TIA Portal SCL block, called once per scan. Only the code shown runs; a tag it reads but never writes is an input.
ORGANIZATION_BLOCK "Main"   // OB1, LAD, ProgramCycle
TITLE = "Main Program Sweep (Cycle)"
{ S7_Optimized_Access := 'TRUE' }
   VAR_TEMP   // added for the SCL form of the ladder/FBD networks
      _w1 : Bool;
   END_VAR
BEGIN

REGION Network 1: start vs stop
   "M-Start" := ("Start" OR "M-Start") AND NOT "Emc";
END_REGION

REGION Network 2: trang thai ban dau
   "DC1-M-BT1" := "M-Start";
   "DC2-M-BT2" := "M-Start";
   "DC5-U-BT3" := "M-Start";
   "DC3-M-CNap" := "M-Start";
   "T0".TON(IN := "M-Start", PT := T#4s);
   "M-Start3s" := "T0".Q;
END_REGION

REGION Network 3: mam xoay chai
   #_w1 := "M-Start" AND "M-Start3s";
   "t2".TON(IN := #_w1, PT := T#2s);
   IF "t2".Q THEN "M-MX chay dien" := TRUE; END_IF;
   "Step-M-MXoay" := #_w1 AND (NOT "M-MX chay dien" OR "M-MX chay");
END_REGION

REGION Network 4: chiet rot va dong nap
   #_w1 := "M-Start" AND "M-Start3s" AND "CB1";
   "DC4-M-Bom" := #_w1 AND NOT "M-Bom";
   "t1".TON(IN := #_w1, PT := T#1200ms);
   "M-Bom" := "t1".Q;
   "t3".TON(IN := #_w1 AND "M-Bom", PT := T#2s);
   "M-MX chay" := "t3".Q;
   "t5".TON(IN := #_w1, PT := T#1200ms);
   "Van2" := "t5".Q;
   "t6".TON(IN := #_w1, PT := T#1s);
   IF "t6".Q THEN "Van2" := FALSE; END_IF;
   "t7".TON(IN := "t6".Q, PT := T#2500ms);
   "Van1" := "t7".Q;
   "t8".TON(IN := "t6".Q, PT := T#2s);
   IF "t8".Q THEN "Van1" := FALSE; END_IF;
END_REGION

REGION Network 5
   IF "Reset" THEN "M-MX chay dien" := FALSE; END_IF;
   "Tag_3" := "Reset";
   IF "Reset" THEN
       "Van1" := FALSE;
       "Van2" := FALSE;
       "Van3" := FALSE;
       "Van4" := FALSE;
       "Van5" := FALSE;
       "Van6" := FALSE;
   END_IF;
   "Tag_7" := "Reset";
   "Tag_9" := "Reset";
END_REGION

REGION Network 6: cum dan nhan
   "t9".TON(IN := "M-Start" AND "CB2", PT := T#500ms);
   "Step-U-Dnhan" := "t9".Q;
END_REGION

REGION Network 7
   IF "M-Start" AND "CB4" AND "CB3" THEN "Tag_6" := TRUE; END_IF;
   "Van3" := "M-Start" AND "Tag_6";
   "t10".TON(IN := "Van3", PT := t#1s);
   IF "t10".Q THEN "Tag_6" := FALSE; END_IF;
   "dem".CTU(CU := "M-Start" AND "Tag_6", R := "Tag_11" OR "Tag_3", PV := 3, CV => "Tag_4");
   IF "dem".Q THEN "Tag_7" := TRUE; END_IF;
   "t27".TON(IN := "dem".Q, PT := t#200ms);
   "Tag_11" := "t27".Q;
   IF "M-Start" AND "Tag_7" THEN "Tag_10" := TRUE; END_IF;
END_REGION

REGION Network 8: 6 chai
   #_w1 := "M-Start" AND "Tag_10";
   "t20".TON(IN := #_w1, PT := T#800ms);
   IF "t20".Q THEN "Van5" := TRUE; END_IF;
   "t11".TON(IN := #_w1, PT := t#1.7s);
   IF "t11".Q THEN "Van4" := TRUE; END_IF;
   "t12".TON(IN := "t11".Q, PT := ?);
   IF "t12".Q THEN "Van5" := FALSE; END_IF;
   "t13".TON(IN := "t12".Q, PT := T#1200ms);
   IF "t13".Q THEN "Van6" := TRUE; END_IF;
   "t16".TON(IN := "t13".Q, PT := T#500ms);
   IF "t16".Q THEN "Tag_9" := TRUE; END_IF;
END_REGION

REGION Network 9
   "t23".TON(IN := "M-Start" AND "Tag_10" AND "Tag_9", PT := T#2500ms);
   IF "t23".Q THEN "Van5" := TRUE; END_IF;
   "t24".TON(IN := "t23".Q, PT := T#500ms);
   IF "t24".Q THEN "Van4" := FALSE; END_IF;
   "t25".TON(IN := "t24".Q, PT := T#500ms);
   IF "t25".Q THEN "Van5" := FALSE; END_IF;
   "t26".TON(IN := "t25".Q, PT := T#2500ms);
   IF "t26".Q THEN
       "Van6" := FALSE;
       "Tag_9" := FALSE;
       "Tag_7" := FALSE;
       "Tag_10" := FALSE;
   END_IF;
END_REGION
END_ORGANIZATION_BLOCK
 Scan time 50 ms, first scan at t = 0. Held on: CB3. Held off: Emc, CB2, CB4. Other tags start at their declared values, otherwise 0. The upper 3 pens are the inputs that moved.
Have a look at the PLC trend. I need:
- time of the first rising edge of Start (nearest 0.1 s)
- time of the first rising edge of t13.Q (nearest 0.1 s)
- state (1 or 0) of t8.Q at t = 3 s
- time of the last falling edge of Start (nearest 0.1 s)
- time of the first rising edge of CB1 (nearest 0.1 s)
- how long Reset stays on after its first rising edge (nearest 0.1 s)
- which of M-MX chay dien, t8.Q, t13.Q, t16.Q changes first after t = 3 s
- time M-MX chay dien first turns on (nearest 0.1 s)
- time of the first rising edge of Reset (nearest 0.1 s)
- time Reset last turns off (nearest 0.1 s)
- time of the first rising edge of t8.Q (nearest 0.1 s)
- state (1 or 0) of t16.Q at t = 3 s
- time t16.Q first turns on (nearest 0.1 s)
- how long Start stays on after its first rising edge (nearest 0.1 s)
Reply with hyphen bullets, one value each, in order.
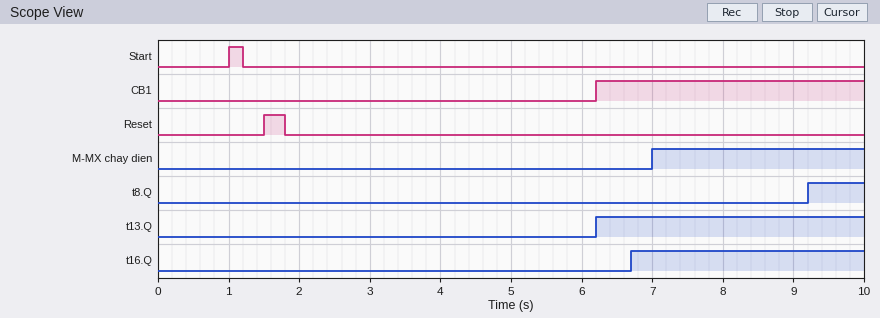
- 1.0 s
- 6.2 s
- 0
- 1.2 s
- 6.2 s
- 0.3 s
- t13.Q
- 7.0 s
- 1.5 s
- 1.8 s
- 9.2 s
- 0
- 6.7 s
- 0.2 s
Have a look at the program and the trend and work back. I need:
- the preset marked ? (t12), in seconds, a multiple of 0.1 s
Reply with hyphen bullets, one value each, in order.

- 1.8 s
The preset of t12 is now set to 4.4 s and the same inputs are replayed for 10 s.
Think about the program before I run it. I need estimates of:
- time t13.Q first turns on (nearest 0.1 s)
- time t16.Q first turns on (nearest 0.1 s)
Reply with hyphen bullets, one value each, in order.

- 8.8 s
- 9.3 s
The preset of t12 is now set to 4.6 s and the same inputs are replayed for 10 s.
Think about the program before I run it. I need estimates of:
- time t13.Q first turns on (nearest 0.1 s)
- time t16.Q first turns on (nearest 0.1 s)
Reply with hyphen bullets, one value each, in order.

- 9.0 s
- 9.5 s
